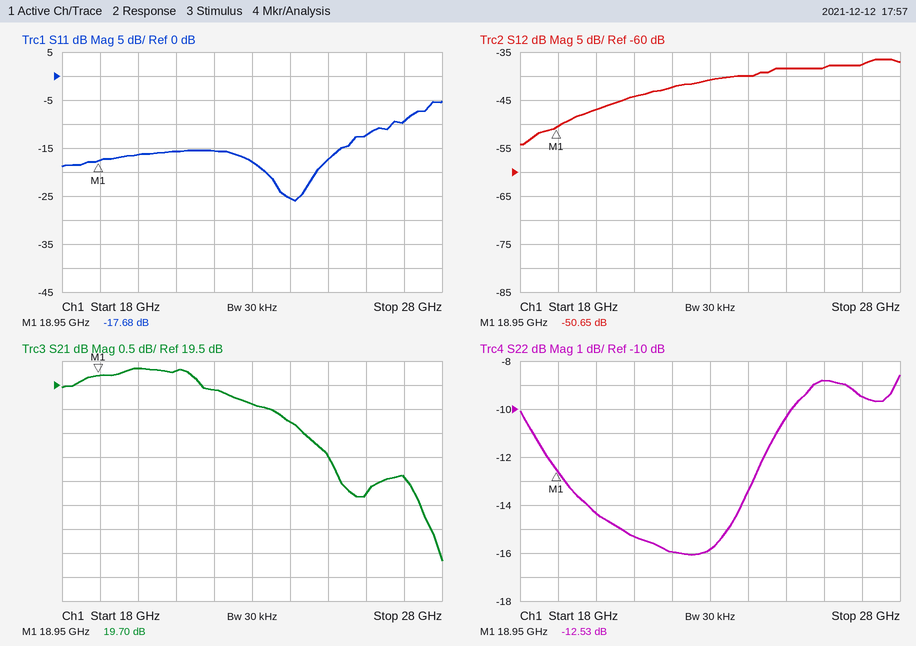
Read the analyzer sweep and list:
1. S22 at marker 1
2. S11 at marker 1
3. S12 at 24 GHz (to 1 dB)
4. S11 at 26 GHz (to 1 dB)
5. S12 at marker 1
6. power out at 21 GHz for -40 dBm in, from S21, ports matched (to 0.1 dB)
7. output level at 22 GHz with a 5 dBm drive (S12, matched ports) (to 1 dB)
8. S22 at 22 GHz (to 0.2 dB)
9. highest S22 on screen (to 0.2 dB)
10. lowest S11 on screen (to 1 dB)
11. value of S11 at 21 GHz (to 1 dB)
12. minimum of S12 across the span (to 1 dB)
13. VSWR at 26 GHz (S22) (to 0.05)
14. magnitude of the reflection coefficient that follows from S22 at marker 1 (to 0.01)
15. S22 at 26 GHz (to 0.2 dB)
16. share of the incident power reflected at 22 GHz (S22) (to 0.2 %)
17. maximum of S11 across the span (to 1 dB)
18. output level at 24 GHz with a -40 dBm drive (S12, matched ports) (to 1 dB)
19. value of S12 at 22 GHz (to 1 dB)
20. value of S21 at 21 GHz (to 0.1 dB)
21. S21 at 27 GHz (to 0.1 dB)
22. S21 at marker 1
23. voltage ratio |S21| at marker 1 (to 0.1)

-12.53 dB
-17.68 dB
-40 dB
-12 dB
-50.65 dB
-20.2 dBm
-37 dBm
-16.0 dB
-8.6 dB
-26 dB
-16 dB
-54 dB
2.15
0.24
-8.8 dB
2.6 %
-5 dB
-80 dBm
-42 dB
19.8 dB
17.6 dB
19.70 dB
9.7
